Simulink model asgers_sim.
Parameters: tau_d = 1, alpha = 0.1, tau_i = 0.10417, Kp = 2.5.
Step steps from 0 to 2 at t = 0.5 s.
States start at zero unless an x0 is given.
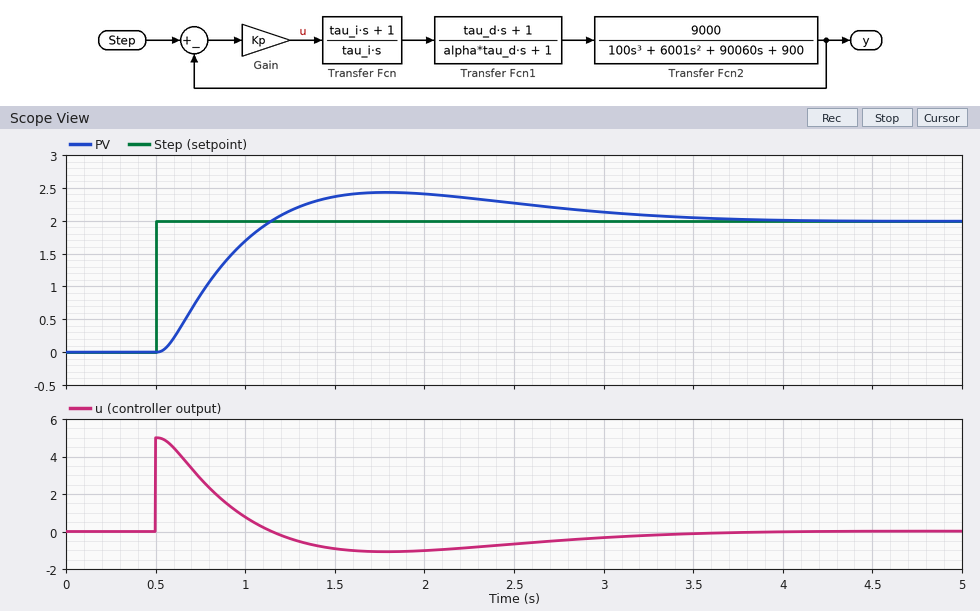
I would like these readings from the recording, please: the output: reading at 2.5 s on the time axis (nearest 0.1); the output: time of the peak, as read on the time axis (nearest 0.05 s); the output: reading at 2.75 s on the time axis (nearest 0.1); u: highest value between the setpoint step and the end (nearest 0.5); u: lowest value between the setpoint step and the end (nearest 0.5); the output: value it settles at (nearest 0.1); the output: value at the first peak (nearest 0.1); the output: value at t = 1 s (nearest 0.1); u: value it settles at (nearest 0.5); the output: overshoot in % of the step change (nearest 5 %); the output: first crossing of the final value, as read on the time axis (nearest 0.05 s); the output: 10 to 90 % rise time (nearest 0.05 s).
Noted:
2.3
1.80 s
2.2
5.0
-1.0
2.0
2.4
1.7
0.0
20 %
1.15 s
0.45 s
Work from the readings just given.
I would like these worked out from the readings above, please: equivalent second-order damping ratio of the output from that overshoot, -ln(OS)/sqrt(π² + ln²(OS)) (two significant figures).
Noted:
0.46
